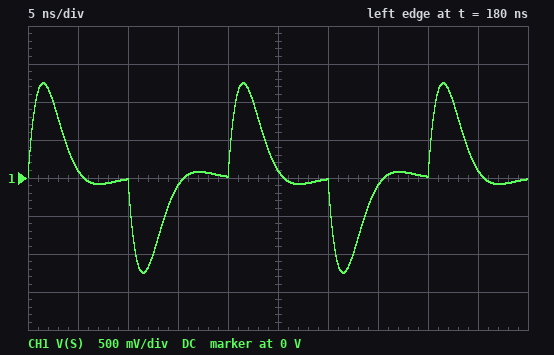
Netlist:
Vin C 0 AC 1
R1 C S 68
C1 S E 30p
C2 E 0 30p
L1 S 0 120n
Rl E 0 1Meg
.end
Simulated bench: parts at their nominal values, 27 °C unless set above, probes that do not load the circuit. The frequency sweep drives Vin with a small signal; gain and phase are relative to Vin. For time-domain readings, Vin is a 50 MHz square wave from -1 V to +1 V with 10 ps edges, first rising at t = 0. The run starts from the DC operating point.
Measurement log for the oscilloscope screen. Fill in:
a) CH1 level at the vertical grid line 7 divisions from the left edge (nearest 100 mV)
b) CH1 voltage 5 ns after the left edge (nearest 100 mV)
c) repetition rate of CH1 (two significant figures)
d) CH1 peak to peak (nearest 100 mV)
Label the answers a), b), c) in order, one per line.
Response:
a) -100 mV
b) 100 mV
c) 50 MHz
d) 2.5 V
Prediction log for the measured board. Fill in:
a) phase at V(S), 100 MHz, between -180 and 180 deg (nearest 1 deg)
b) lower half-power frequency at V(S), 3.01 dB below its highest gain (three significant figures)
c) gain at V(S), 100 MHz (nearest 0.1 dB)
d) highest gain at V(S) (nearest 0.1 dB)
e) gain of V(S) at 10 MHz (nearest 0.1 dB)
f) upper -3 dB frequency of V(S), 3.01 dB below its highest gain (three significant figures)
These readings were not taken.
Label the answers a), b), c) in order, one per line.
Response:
a) 15 deg
b) 64.0 MHz
c) -0.3 dB
d) 0 dB
e) -19.1 dB
f) 220 MHz
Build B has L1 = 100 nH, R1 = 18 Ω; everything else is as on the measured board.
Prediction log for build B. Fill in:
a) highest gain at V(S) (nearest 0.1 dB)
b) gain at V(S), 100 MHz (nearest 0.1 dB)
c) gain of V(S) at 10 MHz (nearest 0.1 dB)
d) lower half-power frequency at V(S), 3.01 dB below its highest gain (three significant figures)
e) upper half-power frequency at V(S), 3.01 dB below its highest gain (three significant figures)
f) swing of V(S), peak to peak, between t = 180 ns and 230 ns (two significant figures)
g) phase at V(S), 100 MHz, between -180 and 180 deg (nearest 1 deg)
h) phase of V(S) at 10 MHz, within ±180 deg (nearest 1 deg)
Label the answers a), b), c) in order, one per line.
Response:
a) 0 dB
b) -0.1 dB
c) -9.6 dB
d) 27.4 MHz
e) 617 MHz
f) 3.1 V
g) 7 deg
h) 71 deg
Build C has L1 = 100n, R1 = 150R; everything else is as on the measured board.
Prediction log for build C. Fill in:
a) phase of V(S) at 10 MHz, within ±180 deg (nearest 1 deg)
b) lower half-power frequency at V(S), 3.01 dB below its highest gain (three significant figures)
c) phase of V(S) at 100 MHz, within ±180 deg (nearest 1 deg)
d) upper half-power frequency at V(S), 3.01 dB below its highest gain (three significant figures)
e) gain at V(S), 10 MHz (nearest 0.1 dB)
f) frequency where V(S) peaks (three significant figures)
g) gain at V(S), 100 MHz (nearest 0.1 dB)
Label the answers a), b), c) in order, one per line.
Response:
a) 88 deg
b) 99.3 MHz
c) 44 deg
d) 170 MHz
e) -27.5 dB
f) 130 MHz
g) -2.9 dB
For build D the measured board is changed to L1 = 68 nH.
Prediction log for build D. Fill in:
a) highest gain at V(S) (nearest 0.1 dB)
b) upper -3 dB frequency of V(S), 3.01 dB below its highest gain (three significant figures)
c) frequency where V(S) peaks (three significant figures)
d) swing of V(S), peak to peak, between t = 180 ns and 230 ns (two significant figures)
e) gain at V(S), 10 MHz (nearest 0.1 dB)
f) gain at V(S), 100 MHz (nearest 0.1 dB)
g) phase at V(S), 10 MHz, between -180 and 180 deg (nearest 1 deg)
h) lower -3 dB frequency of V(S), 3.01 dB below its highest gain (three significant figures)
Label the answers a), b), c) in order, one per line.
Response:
a) 0 dB
b) 254 MHz
c) 158 MHz
d) 2.2 V
e) -24.0 dB
f) -2.8 dB
g) 86 deg
h) 97.8 MHz
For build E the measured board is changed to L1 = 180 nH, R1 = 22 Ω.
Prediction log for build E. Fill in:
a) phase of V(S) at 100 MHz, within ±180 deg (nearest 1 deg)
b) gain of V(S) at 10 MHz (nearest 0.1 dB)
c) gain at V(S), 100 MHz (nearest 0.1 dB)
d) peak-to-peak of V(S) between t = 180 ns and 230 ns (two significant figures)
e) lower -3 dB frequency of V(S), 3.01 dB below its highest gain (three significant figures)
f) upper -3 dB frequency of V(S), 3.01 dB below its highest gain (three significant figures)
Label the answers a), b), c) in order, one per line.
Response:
a) -1 deg
b) -6.7 dB
c) 0 dB
d) 2.8 V
e) 18.7 MHz
f) 501 MHz
